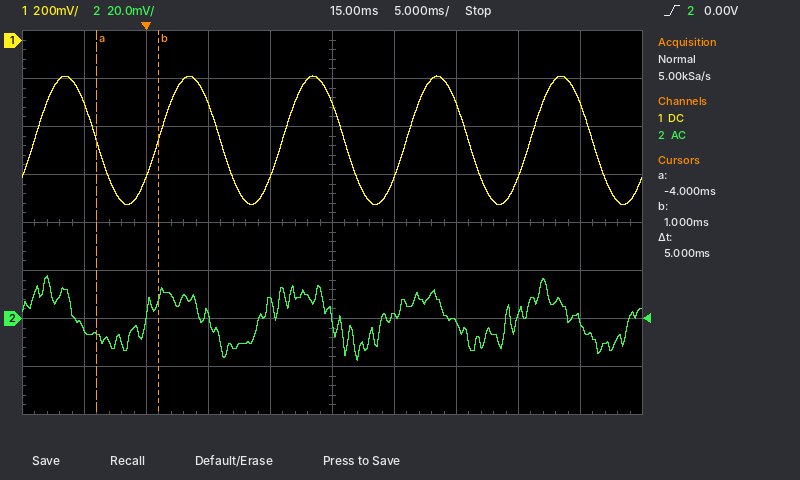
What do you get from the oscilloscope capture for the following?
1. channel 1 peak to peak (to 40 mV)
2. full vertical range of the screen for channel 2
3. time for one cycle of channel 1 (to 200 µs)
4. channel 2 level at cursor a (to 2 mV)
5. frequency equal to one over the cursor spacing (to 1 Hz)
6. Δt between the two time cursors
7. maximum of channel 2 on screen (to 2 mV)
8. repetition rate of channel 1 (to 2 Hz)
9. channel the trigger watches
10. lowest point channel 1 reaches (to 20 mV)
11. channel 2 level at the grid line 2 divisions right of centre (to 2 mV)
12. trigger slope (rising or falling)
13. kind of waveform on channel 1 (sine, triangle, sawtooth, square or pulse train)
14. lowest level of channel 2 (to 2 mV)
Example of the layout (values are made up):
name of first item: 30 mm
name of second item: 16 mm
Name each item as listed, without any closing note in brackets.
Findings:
channel 1 peak to peak: 520 mV
full vertical range of the screen for channel 2: 160 mV
time for one cycle of channel 1: 10.0 ms
channel 2 level at cursor a: -6 mV
frequency equal to one over the cursor spacing: 200 Hz
Δt between the two time cursors: 5 ms
maximum of channel 2 on screen: 18 mV
repetition rate of channel 1: 100 Hz
channel the trigger watches: channel 2
lowest point channel 1 reaches: -680 mV
channel 2 level at the grid line 2 divisions right of centre: -2 mV
trigger slope: rising
kind of waveform on channel 1: sine
lowest level of channel 2: -18 mV
